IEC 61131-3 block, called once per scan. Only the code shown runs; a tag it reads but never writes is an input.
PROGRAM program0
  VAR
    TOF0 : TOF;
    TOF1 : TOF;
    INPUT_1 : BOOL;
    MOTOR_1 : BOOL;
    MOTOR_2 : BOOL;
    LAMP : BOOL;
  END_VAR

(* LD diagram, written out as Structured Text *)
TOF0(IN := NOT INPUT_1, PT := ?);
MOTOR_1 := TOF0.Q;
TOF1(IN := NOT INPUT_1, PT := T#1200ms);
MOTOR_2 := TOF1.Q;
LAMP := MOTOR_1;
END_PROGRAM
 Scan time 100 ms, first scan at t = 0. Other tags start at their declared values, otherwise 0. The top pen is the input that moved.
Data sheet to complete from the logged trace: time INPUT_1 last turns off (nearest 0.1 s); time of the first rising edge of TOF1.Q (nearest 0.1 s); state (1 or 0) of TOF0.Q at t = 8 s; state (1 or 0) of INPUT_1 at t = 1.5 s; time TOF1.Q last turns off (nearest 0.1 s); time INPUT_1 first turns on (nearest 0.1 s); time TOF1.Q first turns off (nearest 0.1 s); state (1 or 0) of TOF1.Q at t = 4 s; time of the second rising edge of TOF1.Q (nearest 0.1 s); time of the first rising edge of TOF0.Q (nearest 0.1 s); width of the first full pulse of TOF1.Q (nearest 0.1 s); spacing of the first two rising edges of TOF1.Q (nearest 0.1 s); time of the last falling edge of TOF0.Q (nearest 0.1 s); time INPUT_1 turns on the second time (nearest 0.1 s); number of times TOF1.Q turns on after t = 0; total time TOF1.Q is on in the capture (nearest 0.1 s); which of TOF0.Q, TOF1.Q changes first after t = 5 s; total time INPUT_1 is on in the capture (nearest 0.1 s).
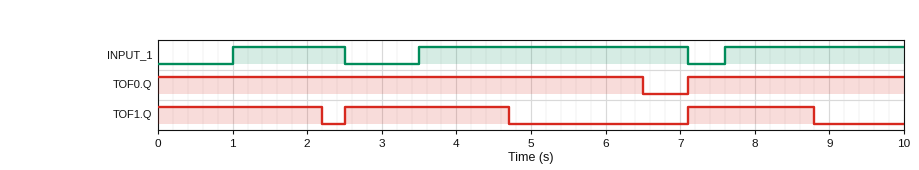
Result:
7.1 s
2.5 s
1
1
8.8 s
1.0 s
2.2 s
1
7.1 s
7.1 s
2.2 s
4.6 s
6.5 s
3.5 s
2
6.1 s
TOF0.Q
7.5 s
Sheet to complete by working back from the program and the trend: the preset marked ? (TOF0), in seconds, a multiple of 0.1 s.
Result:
3.0 s
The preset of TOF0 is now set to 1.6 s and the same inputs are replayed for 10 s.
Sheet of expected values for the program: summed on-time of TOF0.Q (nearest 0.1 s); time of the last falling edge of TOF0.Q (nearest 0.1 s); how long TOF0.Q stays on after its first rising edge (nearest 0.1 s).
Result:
7.2 s
9.2 s
2.1 s
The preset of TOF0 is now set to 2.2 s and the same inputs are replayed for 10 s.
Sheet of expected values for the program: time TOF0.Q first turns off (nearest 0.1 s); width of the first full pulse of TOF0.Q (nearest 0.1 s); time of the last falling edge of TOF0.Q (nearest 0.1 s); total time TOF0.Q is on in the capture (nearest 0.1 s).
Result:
5.7 s
2.7 s
9.8 s
8.4 s
